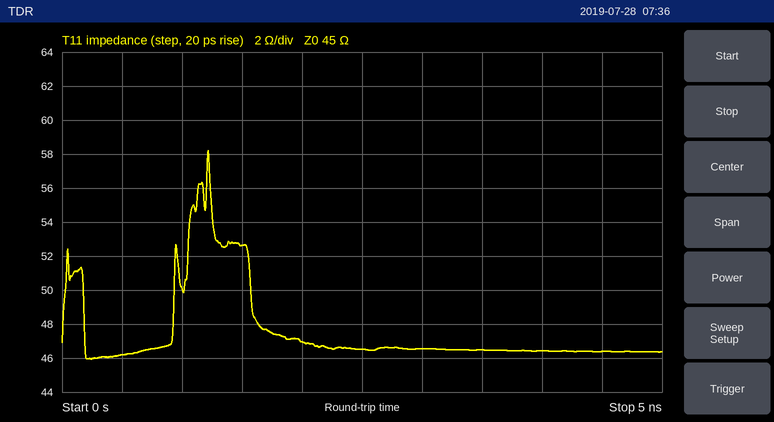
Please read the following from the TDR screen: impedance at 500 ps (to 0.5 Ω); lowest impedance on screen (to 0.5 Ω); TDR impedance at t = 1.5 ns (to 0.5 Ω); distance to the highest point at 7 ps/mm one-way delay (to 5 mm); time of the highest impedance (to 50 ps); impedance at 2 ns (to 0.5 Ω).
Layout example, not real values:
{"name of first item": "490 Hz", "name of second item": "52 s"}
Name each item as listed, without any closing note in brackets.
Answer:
{"impedance at 500 ps": "46.0 Ω", "lowest impedance on screen": "46.0 Ω", "TDR impedance at t = 1.5 ns": "52.5 Ω", "distance to the highest point at 7 ps/mm one-way delay": "85 mm", "time of the highest impedance": "1.20 ns", "impedance at 2 ns": "47.0 Ω"}
